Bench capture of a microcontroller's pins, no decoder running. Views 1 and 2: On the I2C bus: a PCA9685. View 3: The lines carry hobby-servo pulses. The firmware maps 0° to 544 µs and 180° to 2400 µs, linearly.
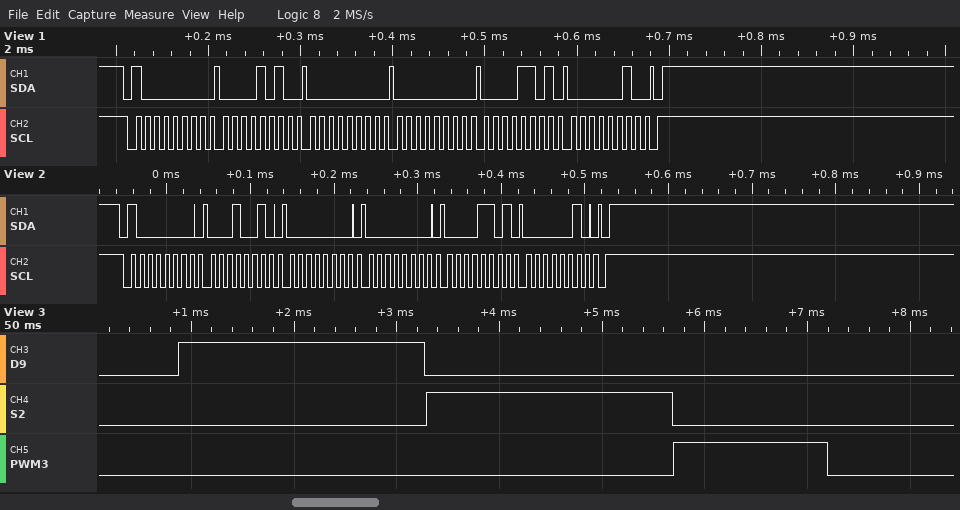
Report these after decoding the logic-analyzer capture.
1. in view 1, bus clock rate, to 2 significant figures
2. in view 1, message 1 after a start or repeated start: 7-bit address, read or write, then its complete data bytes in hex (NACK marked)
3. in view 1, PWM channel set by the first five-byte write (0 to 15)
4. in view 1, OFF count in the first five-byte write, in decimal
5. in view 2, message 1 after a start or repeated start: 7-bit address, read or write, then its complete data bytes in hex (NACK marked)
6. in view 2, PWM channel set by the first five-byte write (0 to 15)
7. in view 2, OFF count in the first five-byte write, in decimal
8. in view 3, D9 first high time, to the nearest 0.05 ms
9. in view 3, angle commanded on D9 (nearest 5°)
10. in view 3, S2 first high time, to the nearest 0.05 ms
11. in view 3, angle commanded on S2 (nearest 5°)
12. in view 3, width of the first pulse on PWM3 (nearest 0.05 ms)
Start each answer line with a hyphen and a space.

- 100 kHz
- 0x40 write: 0A 00 00 0D 02
- 1
- 525
- 0x40 write: 12 00 00 0D 02
- 3
- 525
- 2.40 ms
- 180°
- 2.40 ms
- 180°
- 1.50 ms
